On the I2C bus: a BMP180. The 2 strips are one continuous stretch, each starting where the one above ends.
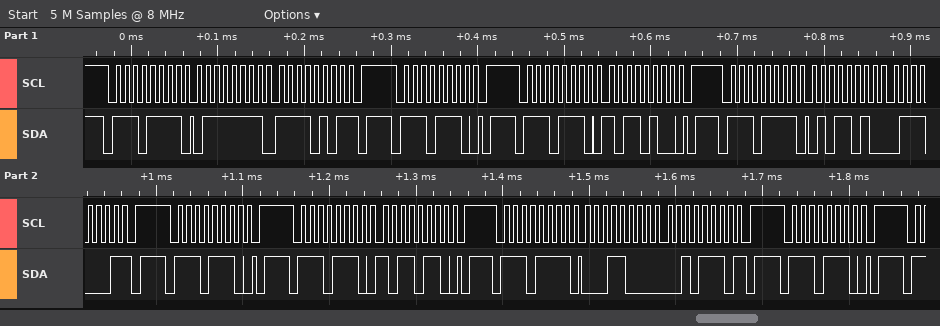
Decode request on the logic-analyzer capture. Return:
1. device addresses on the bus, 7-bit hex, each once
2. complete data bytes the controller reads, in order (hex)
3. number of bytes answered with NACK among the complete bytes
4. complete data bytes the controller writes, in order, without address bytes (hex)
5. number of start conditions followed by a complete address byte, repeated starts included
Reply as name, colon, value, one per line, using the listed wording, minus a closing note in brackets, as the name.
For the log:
device addresses on the bus, 7-bit hex, each once: 0x77
complete data bytes the controller reads, in order: 7F F5 5A 71 18 2E
number of bytes answered with NACK among the complete bytes: 3
complete data bytes the controller writes, in order, without address bytes: B4 B6
number of start conditions followed by a complete address byte, repeated starts included: 8
